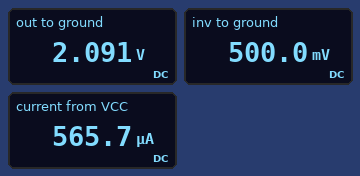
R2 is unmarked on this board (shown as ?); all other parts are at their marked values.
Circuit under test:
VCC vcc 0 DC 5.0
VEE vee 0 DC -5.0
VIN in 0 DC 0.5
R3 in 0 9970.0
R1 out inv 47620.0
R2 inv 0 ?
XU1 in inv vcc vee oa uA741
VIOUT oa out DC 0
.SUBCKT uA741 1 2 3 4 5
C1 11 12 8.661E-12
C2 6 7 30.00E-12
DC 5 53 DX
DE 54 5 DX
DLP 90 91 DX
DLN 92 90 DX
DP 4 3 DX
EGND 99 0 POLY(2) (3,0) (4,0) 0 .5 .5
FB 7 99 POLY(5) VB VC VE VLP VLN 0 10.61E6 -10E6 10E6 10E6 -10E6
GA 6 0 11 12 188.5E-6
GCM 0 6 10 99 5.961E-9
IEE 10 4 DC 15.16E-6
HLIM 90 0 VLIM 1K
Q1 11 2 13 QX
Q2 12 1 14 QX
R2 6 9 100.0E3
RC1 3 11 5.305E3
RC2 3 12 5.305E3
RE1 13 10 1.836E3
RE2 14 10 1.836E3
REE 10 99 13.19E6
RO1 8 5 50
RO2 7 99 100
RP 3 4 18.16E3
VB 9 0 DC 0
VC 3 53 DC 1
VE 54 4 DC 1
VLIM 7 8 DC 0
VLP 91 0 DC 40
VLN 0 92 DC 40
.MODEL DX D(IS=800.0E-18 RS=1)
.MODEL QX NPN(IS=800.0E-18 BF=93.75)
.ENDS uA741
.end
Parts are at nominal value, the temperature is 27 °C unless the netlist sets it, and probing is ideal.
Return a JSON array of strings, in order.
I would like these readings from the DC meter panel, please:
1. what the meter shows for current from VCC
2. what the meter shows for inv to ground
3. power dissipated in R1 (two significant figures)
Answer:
["565.7 µA", "500.0 mV", "53 µW"]
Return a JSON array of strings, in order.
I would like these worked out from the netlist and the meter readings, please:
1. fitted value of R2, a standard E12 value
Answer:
["15 kΩ"]
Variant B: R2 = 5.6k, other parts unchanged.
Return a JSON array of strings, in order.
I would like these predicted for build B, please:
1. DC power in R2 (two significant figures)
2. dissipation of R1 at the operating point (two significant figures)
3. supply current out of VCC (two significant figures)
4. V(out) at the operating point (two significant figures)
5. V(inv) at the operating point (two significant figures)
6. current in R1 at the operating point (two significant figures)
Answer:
["41 µW", "350 µW", "560 µA", "4.6 V", "480 mV", "86 µA"]
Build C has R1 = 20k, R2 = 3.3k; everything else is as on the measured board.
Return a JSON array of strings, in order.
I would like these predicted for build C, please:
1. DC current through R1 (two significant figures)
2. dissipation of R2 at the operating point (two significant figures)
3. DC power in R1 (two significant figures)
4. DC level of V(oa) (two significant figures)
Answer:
["150 µA", "76 µW", "460 µW", "3.5 V"]
